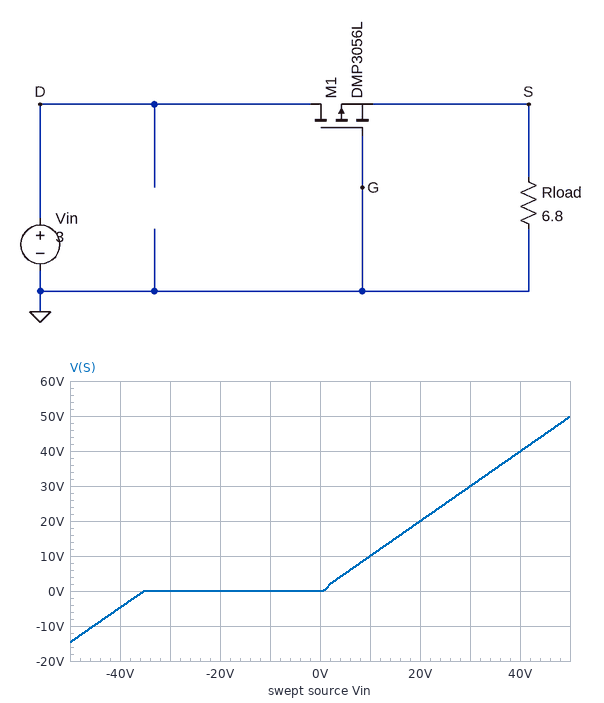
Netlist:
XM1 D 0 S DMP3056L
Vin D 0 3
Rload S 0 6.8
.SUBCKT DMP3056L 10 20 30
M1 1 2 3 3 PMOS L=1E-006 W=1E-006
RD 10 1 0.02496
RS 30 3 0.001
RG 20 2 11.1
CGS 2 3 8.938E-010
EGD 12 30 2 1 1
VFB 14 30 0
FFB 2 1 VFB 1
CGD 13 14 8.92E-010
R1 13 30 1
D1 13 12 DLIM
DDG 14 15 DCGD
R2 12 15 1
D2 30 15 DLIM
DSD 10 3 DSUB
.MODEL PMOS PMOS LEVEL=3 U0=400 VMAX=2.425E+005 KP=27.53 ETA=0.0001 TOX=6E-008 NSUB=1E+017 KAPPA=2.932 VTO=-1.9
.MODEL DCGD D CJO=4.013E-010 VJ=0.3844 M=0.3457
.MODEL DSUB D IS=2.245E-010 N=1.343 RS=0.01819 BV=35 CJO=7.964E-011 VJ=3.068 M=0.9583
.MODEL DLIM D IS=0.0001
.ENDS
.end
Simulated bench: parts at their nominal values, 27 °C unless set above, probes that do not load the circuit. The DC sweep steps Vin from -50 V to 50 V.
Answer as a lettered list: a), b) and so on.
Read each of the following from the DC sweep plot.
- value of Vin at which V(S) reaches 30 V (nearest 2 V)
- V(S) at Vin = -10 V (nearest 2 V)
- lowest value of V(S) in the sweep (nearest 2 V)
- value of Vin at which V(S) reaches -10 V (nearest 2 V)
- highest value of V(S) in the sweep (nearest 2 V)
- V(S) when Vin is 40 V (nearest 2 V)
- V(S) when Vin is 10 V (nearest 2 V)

a) 30 V
b) 0 V
c) -14 V
d) -46 V
e) 50 V
f) 40 V
g) 10 V
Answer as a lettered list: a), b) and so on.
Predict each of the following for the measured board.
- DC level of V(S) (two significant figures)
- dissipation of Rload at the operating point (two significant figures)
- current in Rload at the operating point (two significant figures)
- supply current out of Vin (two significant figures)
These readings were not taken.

a) 3.0 V
b) 1.3 W
c) 440 mA
d) 440 mA
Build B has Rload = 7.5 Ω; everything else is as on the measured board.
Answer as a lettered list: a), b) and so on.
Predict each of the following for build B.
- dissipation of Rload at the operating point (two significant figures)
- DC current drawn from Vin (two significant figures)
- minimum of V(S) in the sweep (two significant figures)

a) 1.2 W
b) 400 mA
c) -15 V
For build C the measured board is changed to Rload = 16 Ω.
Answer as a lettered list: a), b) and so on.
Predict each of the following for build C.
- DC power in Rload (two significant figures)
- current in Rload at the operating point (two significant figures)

a) 560 mW
b) 190 mA
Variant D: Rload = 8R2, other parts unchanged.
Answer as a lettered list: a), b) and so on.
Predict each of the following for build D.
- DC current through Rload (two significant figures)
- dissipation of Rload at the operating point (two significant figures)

a) 360 mA
b) 1.1 W
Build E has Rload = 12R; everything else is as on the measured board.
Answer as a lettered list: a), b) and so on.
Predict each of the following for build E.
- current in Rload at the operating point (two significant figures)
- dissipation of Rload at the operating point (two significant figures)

a) 250 mA
b) 740 mW
